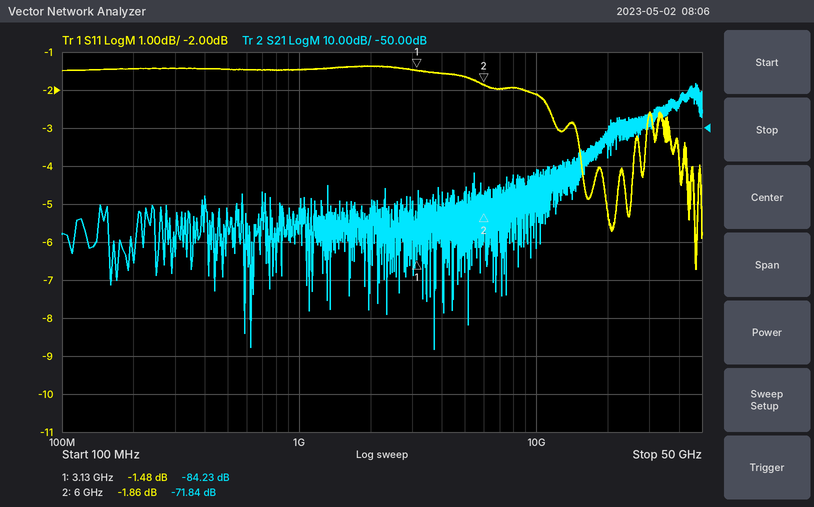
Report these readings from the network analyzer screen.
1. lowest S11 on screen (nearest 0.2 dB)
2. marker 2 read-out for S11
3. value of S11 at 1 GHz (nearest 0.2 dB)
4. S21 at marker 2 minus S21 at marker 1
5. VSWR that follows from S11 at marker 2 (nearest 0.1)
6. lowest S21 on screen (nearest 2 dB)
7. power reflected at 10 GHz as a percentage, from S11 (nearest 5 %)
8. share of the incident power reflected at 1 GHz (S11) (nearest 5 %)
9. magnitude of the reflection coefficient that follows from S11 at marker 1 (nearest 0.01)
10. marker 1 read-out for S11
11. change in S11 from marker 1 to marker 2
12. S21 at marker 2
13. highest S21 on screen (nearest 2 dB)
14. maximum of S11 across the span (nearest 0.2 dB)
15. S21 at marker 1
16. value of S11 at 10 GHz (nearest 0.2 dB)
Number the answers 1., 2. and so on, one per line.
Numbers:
1. -6.8 dB
2. -1.86 dB
3. -1.4 dB
4. 12.39 dB
5. 9.4
6. -108 dB
7. 60 %
8. 70 %
9. 0.84
10. -1.48 dB
11. -0.38 dB
12. -71.84 dB
13. -38 dB
14. -1.4 dB
15. -84.23 dB
16. -2.2 dB
